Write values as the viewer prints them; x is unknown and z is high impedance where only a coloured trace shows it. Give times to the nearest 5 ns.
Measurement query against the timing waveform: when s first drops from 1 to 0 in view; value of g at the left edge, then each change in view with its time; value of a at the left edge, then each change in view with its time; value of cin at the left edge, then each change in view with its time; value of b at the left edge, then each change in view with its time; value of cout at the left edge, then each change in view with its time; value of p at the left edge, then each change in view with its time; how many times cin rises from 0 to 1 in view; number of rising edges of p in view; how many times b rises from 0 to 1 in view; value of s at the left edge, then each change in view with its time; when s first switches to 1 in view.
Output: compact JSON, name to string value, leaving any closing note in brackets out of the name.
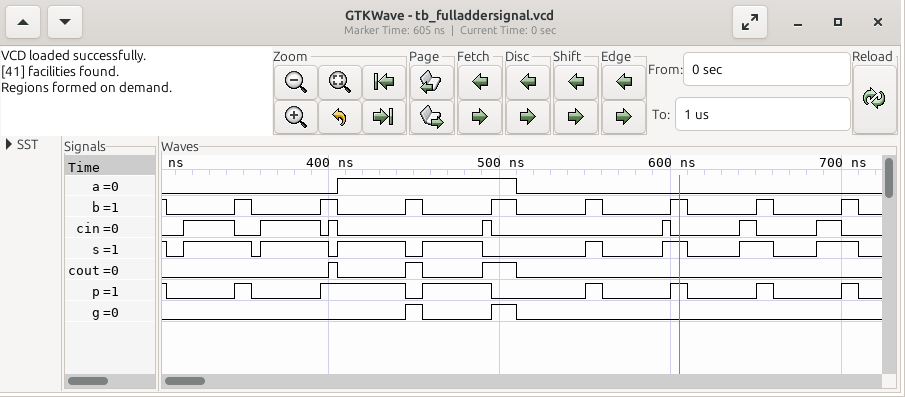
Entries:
{"when s first drops from 1 to 0 in view": "305 ns", "value of g at the left edge, then each change in view with its time": "0, 1 at 445 ns, 0 at 455 ns, 1 at 495 ns, 0 at 510 ns", "value of a at the left edge, then each change in view with its time": "0, 1 at 405 ns, 0 at 510 ns", "value of cin at the left edge, then each change in view with its time": "0, 1 at 315 ns, 0 at 345 ns, 1 at 360 ns, 0 at 395 ns, 1 at 400 ns, 0 at 405 ns, 1 at 490 ns, 0 at 495 ns, 1 at 595 ns, 0 at 600 ns, 1 at 640 ns, 0 at 650 ns, 1 at 685 ns, 0 at 700 ns", "value of b at the left edge, then each change in view with its time": "1, 0 at 305 ns, 1 at 345 ns, 0 at 355 ns, 1 at 395 ns, 0 at 405 ns, 1 at 445 ns, 0 at 455 ns, 1 at 495 ns, 0 at 510 ns, 1 at 550 ns, 0 at 560 ns, 1 at 600 ns, 0 at 610 ns, 1 at 650 ns, 0 at 660 ns, 1 at 700 ns, 0 at 710 ns", "value of cout at the left edge, then each change in view with its time": "0, 1 at 400 ns, 0 at 405 ns, 1 at 445 ns, 0 at 455 ns, 1 at 490 ns, 0 at 510 ns", "value of p at the left edge, then each change in view with its time": "1, 0 at 305 ns, 1 at 345 ns, 0 at 355 ns, 1 at 395 ns, 0 at 445 ns, 1 at 455 ns, 0 at 495 ns, 1 at 550 ns, 0 at 560 ns, 1 at 600 ns, 0 at 610 ns, 1 at 650 ns, 0 at 660 ns, 1 at 700 ns, 0 at 710 ns", "how many times cin rises from 0 to 1 in view": "7", "number of rising edges of p in view": "7", "how many times b rises from 0 to 1 in view": "8", "value of s at the left edge, then each change in view with its time": "1, 0 at 305 ns, 1 at 315 ns, 0 at 355 ns, 1 at 360 ns, 0 at 400 ns, 1 at 405 ns, 0 at 445 ns, 1 at 455 ns, 0 at 490 ns, 1 at 550 ns, 0 at 560 ns, 1 at 595 ns, 0 at 610 ns, 1 at 640 ns, 0 at 660 ns, 1 at 685 ns, 0 at 710 ns", "when s first switches to 1 in view": "315 ns"}
